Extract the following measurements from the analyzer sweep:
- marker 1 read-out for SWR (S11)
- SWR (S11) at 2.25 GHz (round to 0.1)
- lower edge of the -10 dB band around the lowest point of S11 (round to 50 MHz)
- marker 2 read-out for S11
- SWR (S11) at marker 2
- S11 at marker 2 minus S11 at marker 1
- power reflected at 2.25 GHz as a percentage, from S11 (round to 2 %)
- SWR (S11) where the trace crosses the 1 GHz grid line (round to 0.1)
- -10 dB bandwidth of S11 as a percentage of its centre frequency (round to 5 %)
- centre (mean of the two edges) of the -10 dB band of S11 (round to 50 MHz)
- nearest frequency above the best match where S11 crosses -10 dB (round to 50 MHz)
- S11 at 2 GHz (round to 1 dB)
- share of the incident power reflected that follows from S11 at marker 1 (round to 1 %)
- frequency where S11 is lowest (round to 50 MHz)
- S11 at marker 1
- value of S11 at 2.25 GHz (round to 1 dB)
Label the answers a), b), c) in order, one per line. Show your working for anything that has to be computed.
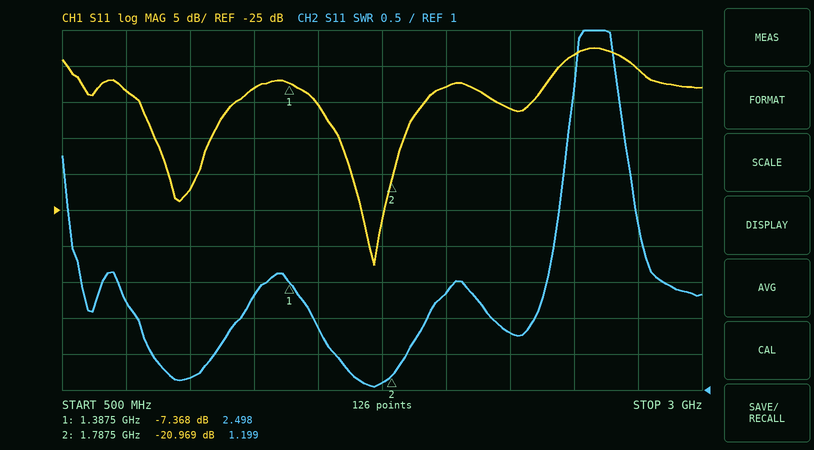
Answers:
a) 2.498
b) 1.8
c) 1.50 GHz
d) -20.969 dB
e) 1.199
f) -20.969 − (-7.368) = -13.601 dB
g) 10^(-11/10) ≈ 8 %
h) 1.2
i) 400 MHz / 1.7 GHz ≈ 23.5 %, so 25 % to the nearest 5 %
j) 1.70 GHz
k) 1.90 GHz
l) -8 dB
m) 10^(-7.368/10) ≈ 18 %
n) 1.70 GHz
o) -7.368 dB
p) -11 dB
